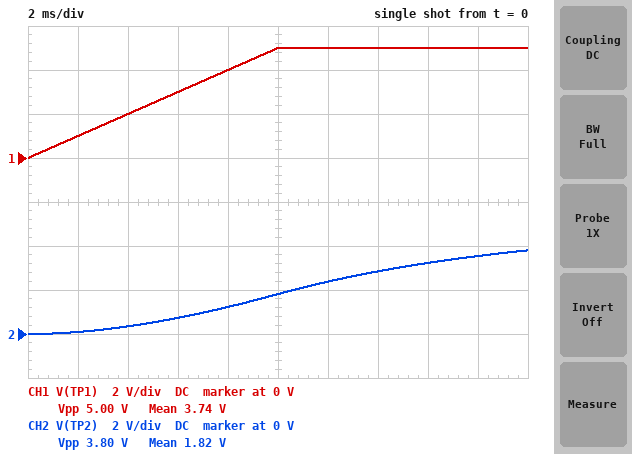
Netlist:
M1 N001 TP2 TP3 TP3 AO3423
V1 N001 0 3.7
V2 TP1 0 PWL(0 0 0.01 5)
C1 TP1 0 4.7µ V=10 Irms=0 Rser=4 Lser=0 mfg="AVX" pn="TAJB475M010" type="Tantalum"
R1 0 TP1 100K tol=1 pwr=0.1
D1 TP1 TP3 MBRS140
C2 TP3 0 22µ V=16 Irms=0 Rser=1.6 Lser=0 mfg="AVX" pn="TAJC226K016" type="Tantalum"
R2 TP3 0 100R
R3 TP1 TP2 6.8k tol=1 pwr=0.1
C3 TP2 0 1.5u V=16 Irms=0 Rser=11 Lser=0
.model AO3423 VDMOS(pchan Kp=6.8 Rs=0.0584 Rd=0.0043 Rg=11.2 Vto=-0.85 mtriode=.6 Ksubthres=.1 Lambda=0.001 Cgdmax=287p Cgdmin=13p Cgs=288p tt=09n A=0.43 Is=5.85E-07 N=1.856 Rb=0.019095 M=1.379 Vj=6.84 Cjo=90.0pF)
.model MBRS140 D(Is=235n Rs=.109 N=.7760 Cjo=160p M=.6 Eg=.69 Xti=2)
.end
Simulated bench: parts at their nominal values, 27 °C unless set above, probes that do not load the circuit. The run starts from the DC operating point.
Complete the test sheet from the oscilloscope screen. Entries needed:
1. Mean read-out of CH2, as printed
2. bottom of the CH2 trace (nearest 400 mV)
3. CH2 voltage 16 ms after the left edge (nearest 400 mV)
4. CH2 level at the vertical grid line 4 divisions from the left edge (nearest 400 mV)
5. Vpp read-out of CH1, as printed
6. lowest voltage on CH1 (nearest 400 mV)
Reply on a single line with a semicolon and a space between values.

1.82 V; 0 V; 3.2 V; 1.2 V; 5.00 V; 0 V
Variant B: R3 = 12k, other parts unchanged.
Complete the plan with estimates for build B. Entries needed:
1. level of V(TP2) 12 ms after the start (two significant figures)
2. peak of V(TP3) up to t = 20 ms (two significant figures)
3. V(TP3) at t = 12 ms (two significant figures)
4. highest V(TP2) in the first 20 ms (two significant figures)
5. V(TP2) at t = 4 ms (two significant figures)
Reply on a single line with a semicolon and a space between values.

1.6 V; 4.5 V; 4.3 V; 2.8 V; 210 mV
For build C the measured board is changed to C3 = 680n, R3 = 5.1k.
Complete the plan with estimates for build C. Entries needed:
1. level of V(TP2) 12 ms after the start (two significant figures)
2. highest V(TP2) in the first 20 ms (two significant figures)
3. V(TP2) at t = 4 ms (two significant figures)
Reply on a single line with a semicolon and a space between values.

4.1 V; 4.9 V; 810 mV
